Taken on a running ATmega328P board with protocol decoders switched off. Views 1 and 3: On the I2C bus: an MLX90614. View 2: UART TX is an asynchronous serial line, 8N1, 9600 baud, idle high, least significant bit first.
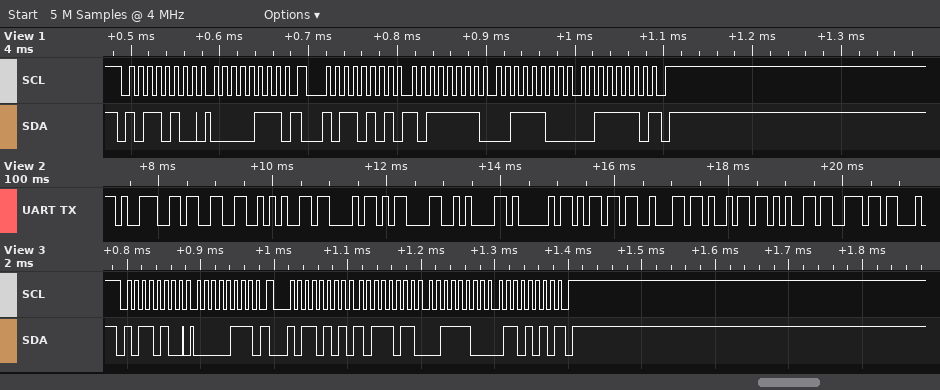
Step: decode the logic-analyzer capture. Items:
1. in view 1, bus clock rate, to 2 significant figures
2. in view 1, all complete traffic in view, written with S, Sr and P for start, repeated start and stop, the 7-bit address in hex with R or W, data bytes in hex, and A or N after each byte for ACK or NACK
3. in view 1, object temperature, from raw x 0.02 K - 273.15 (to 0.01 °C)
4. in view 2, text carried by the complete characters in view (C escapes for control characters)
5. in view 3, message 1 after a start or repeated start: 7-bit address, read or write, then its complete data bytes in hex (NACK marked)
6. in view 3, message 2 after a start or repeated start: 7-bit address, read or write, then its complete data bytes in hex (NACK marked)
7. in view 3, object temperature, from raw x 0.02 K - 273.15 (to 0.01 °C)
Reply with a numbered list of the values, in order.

1. 100 kHz
2. S 5AW A 07 A Sr 5AR A BF A 3C A 3E N P
3. 37.87 °C
4. "93*C\r\nAmbien"
5. 0x5A write: 07
6. 0x5A read: BB 3C 6A NACK
7. 37.79 °C
